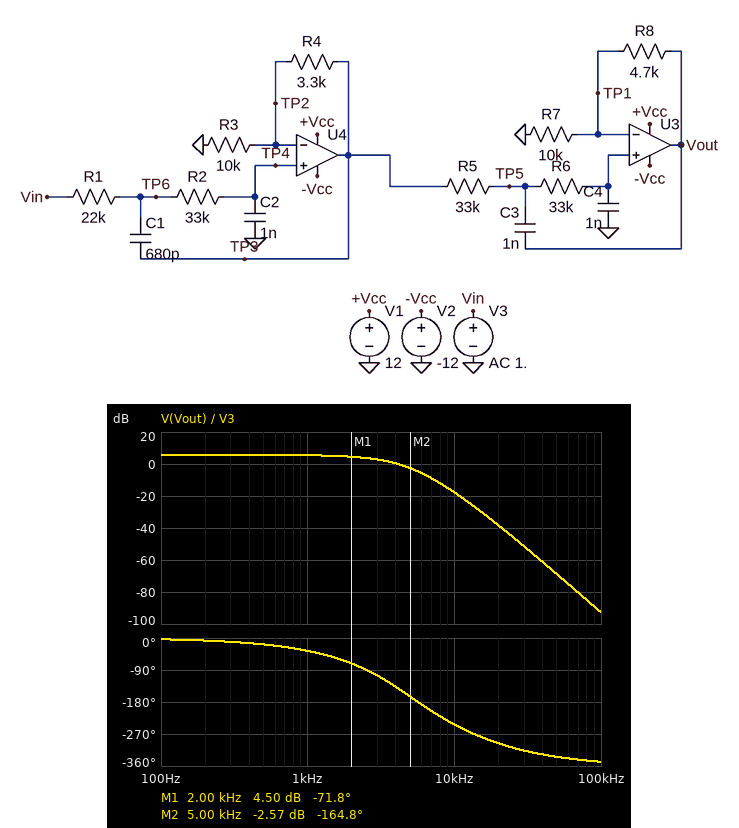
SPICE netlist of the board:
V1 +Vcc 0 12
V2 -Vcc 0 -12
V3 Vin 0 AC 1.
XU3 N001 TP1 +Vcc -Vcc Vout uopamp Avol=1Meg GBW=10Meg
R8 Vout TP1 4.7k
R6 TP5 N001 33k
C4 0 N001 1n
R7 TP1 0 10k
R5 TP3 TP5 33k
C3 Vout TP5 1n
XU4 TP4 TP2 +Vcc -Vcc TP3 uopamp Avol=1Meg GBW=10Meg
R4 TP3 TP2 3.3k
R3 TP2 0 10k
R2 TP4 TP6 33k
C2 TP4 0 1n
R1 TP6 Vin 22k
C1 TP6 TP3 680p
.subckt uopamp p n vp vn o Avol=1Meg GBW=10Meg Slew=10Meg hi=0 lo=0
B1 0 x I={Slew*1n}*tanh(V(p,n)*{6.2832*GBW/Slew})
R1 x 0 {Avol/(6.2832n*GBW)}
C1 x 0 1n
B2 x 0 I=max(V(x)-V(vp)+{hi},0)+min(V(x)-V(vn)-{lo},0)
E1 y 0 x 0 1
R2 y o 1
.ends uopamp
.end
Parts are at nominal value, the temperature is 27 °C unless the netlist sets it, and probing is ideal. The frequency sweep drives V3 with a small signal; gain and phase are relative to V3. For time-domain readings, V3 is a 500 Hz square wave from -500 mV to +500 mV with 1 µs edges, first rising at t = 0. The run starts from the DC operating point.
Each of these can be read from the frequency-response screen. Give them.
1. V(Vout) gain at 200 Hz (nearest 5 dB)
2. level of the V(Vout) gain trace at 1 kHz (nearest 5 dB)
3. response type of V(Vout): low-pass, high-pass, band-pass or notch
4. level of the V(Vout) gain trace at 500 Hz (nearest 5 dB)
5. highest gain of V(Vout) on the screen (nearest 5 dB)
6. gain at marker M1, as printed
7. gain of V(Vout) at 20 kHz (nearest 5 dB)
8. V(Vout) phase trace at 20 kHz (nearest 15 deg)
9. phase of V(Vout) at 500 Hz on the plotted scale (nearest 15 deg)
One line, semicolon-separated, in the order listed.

5 dB; 5 dB; low-pass; 5 dB; 5 dB; 4.50 dB; -40 dB; -300 deg; -15 deg
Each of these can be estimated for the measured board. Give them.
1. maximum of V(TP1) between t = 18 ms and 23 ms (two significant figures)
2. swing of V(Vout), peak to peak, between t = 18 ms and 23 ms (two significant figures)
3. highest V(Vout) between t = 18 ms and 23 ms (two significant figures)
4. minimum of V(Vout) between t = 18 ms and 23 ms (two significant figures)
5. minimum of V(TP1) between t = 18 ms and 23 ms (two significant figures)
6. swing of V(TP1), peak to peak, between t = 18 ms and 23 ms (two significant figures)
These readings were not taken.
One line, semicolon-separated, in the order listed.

670 mV; 2.0 V; 980 mV; -980 mV; -670 mV; 1.3 V
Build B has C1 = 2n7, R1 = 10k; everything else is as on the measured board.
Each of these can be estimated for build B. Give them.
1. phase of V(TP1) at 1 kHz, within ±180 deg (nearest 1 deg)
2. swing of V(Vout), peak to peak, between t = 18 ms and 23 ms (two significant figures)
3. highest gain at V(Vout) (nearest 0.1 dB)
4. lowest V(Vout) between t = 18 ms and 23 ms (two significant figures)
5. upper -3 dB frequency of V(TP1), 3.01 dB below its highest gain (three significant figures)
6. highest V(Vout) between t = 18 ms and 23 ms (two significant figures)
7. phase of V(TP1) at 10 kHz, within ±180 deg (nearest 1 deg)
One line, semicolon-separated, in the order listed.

-31 deg; 2.3 V; 5.9 dB; -1.1 V; 4.42 kHz; 1.1 V; 84 deg
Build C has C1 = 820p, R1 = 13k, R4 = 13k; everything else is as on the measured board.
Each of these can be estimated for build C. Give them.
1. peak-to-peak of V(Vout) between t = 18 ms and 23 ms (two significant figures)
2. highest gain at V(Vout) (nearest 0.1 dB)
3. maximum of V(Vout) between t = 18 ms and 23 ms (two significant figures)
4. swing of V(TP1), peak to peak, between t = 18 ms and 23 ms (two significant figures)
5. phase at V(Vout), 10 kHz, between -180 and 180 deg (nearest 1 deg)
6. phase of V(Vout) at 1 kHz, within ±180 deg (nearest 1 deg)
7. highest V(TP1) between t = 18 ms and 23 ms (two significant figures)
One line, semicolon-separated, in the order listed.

3.5 V; 10.6 dB; 1.8 V; 2.4 V; 123 deg; -30 deg; 1.2 V
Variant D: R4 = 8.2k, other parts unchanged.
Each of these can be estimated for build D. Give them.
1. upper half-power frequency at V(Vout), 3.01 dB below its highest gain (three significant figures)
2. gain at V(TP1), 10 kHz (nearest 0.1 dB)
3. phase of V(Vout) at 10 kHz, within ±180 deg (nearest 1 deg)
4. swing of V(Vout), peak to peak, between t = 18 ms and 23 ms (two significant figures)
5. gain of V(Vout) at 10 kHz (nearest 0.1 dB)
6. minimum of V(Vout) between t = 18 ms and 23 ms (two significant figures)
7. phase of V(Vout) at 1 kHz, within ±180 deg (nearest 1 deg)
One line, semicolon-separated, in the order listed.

3.37 kHz; -17.1 dB; 114 deg; 2.7 V; -13.8 dB; -1.4 V; -34 deg
